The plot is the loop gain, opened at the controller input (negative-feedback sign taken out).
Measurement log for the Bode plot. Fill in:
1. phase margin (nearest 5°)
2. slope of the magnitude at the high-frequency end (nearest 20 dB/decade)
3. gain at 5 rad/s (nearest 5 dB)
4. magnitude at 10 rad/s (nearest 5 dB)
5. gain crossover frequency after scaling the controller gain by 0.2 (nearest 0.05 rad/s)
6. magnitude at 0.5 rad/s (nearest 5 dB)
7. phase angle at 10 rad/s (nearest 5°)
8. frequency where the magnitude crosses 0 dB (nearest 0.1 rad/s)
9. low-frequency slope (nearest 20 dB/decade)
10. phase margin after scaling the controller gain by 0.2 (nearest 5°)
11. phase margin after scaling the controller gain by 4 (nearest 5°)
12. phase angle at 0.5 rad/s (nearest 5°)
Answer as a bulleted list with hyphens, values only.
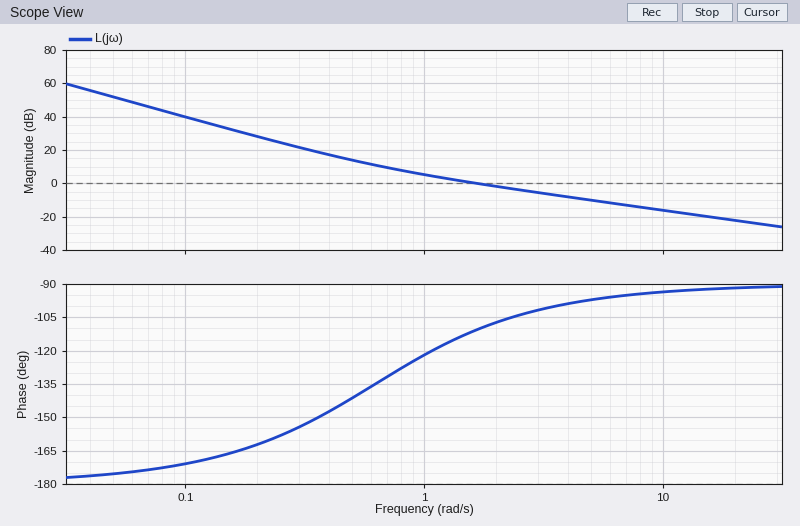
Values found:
- 70°
- -20 dB/decade
- -10 dB
- -15 dB
- 0.50 rad/s
- 15 dB
- -95°
- 1.7 rad/s
- -40 dB/decade
- 40°
- 85°
- -140°
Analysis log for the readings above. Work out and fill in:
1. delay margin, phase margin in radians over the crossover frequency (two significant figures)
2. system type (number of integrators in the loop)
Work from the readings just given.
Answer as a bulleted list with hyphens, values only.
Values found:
- 0.72 s
- 2
